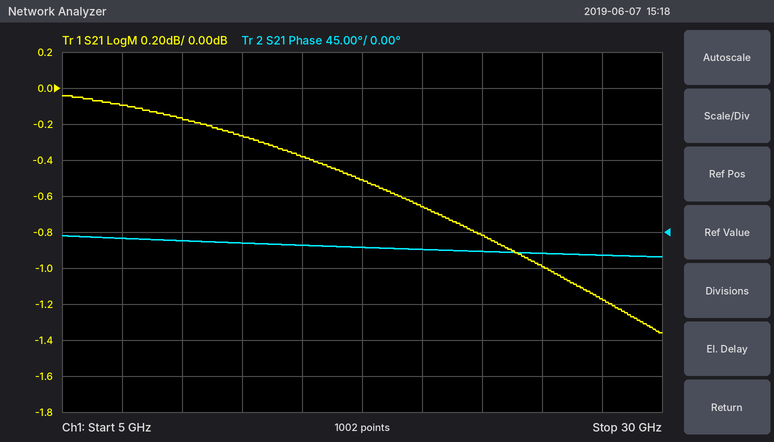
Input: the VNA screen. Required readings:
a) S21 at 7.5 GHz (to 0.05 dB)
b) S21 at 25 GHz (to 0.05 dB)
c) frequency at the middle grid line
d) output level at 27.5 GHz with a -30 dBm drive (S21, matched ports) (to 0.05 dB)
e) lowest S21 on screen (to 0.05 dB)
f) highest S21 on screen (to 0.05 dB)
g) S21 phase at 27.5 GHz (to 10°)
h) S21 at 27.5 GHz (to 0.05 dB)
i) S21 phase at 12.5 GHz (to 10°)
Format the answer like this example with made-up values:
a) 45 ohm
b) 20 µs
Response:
a) -0.10 dB
b) -1.00 dB
c) 17.5 GHz
d) -31.15 dBm
e) -1.35 dB
f) -0.05 dB
g) -30°
h) -1.15 dB
i) -10°
